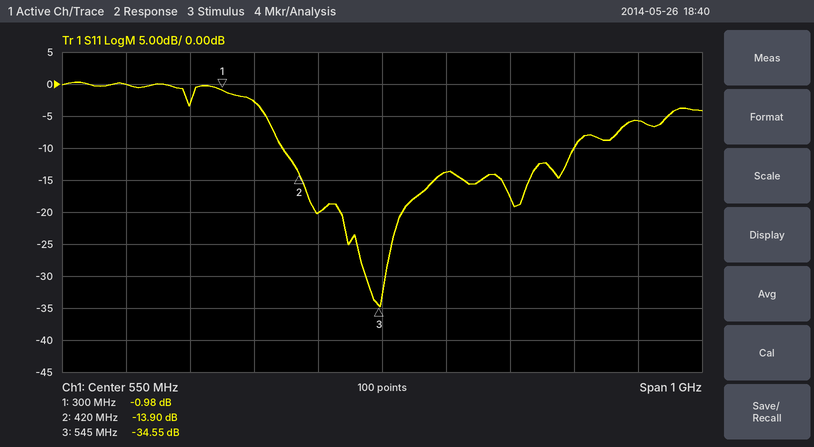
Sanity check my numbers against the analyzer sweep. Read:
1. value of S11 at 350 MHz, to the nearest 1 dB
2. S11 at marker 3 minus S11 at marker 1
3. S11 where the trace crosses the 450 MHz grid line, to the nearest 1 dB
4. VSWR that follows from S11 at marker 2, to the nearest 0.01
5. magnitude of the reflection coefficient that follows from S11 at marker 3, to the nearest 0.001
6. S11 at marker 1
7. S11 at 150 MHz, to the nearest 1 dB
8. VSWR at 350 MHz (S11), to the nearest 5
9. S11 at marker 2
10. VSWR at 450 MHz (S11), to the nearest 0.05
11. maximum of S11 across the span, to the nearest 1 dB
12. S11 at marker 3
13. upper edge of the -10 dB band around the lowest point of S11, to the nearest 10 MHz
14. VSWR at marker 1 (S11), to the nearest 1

-3 dB
-33.57 dB
-20 dB
1.51
0.019
-0.98 dB
0 dB
5
-13.90 dB
1.20
0 dB
-34.55 dB
850 MHz
18
